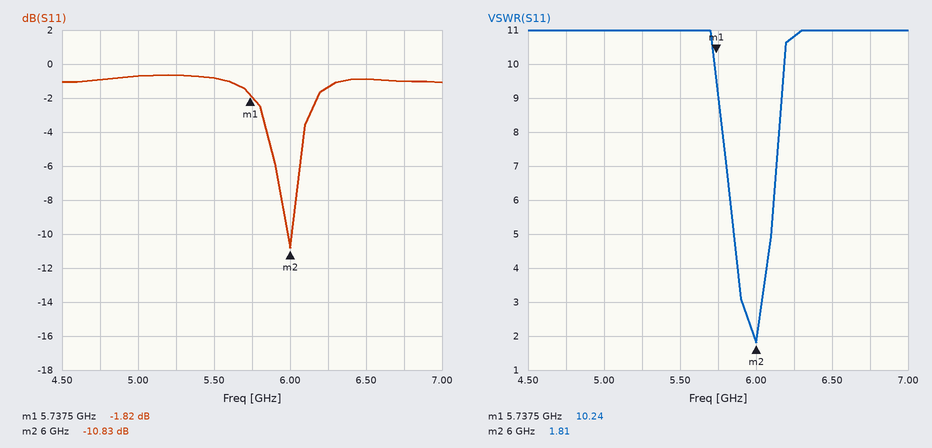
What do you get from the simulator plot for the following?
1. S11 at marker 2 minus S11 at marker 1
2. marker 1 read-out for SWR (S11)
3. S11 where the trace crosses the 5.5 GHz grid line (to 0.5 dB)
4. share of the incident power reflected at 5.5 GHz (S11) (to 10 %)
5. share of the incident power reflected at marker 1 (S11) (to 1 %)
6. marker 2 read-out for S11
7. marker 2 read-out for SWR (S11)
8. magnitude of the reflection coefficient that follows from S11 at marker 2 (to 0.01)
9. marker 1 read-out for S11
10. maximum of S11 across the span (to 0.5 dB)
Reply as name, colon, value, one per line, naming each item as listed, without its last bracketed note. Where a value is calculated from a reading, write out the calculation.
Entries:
S11 at marker 2 minus S11 at marker 1: -10.83 − (-1.82) = -9.01 dB
marker 1 read-out for SWR: 10.24
S11 where the trace crosses the 5.5 GHz grid line: -1.0 dB
share of the incident power reflected at 5.5 GHz (S11): 10^(-1/10) ≈ 79.4 %, so 80 % to the nearest 10 %
share of the incident power reflected at marker 1 (S11): 10^(-1.82/10) ≈ 66 %
marker 2 read-out for S11: -10.83 dB
marker 2 read-out for SWR: 1.81
magnitude of the reflection coefficient that follows from S11 at marker 2: 10^(-10.83/20) ≈ 0.29
marker 1 read-out for S11: -1.82 dB
maximum of S11 across the span: -0.5 dB
